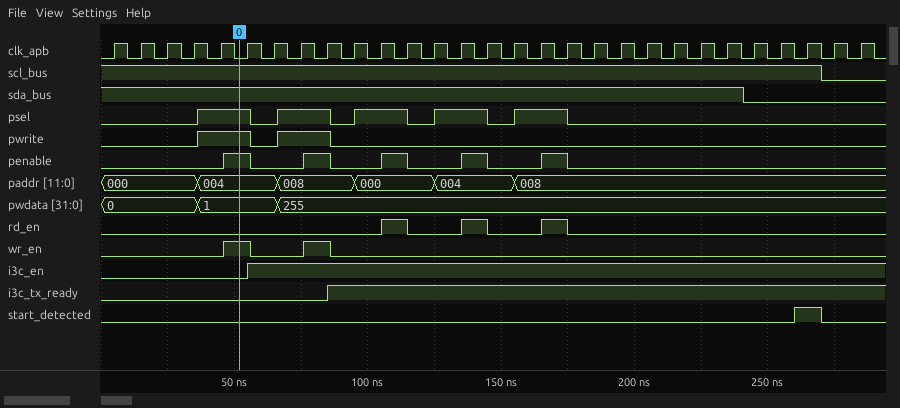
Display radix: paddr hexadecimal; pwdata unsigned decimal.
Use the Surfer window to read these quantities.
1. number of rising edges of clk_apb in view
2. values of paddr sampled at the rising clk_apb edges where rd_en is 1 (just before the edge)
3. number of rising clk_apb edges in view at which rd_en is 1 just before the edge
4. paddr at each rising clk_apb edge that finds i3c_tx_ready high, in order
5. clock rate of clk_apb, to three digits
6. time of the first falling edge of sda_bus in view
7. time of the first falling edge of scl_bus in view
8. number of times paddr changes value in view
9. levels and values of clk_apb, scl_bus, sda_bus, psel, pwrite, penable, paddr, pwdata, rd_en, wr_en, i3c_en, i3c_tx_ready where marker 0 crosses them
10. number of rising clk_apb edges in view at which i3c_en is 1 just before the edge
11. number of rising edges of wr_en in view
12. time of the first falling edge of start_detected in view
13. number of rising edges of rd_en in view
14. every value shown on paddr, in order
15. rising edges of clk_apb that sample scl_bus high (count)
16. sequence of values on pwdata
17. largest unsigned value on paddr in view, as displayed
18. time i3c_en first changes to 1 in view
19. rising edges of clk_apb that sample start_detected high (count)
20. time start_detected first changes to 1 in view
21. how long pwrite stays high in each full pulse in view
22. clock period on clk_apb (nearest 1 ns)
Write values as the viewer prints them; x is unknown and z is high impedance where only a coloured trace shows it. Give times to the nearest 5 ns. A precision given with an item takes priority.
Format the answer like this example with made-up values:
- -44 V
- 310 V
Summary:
- 29
- 000, 004, 008
- 3
- 008, 000, 000, 000, 004, 004, 004, 008, 008, 008, 008, 008, 008, 008, 008, 008, 008, 008, 008, 008
- 100 MHz
- 240 ns
- 270 ns
- 5
- clk_apb=0, scl_bus=1, sda_bus=1, psel=1, pwrite=1, penable=1, paddr=004, pwdata=1, rd_en=0, wr_en=1, i3c_en=0, i3c_tx_ready=0
- 23
- 2
- 270 ns
- 3
- 000, 004, 008, 000, 004, 008
- 27
- 0, 1, 255
- 008
- 55 ns
- 1
- 260 ns
- 20 ns, 20 ns
- 10 ns
